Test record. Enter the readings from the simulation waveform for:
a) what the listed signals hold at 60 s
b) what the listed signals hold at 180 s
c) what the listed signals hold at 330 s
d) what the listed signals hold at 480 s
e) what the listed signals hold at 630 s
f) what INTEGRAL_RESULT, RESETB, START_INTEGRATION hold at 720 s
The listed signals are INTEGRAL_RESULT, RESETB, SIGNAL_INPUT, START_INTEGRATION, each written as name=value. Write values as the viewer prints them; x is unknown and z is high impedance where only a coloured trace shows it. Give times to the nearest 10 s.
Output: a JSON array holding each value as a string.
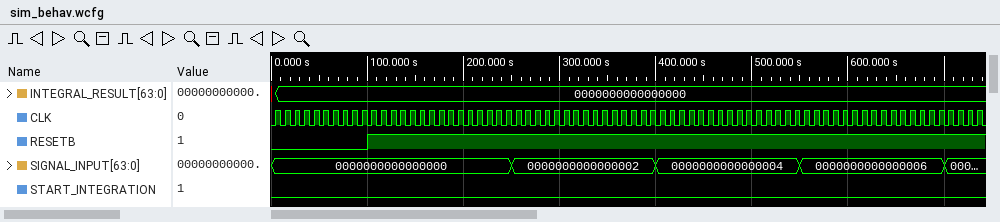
["INTEGRAL_RESULT=0000000000000000, RESETB=0, SIGNAL_INPUT=0000000000000000, START_INTEGRATION=0", "INTEGRAL_RESULT=0000000000000000, RESETB=1, SIGNAL_INPUT=0000000000000000, START_INTEGRATION=0", "INTEGRAL_RESULT=0000000000000000, RESETB=1, SIGNAL_INPUT=0000000000000002, START_INTEGRATION=0", "INTEGRAL_RESULT=0000000000000000, RESETB=1, SIGNAL_INPUT=0000000000000004, START_INTEGRATION=0", "INTEGRAL_RESULT=0000000000000000, RESETB=1, SIGNAL_INPUT=0000000000000006, START_INTEGRATION=0", "INTEGRAL_RESULT=0000000000000000, RESETB=1, START_INTEGRATION=0"]
